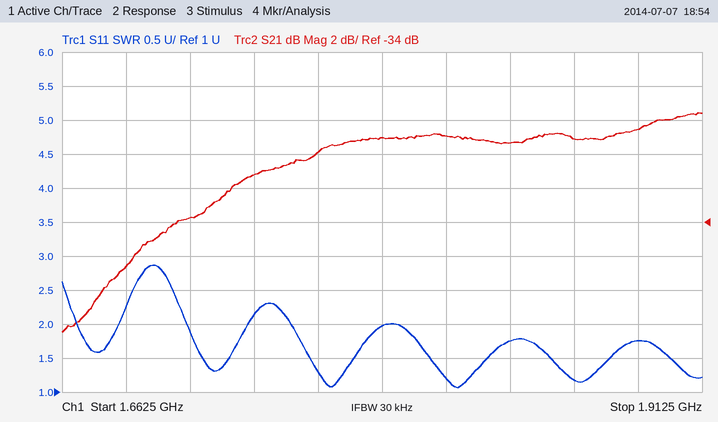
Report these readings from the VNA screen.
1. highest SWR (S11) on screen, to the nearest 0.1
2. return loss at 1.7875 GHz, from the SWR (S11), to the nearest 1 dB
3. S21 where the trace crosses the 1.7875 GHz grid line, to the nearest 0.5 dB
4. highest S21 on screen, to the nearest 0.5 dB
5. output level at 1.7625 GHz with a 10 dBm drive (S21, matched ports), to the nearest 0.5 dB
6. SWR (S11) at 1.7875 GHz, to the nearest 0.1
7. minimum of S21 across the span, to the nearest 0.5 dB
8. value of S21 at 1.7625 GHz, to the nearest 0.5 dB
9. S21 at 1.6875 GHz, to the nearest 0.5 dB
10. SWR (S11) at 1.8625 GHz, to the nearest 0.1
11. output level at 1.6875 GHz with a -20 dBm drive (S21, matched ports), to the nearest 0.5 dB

2.9
10 dB
-29.0 dB
-27.5 dB
-20.0 dBm
2.0
-40.5 dB
-30.0 dB
-36.5 dB
1.2
-56.5 dBm
